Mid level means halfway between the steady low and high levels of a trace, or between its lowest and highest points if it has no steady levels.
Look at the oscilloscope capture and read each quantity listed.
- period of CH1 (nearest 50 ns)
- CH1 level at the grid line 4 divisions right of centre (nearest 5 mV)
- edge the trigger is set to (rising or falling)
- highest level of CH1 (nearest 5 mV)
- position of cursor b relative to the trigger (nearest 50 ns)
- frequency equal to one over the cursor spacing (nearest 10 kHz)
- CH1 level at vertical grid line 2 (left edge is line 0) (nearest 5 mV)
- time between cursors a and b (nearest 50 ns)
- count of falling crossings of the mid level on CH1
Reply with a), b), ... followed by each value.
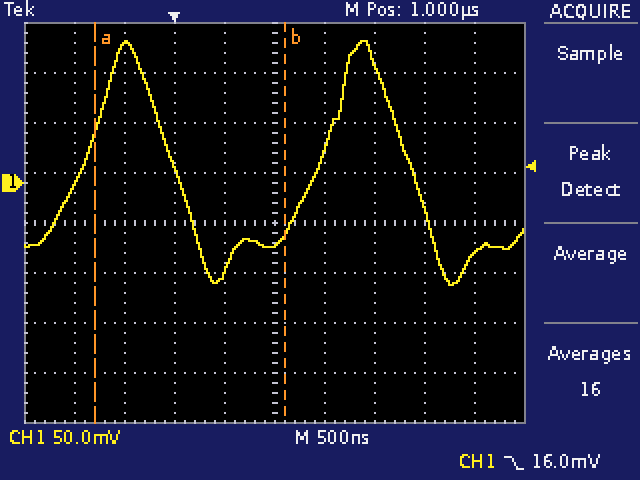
a) 2.35 µs
b) -70 mV
c) falling
d) 140 mV
e) +1.10 µs
f) 530 kHz
g) 140 mV
h) 1.90 µs
i) 2
